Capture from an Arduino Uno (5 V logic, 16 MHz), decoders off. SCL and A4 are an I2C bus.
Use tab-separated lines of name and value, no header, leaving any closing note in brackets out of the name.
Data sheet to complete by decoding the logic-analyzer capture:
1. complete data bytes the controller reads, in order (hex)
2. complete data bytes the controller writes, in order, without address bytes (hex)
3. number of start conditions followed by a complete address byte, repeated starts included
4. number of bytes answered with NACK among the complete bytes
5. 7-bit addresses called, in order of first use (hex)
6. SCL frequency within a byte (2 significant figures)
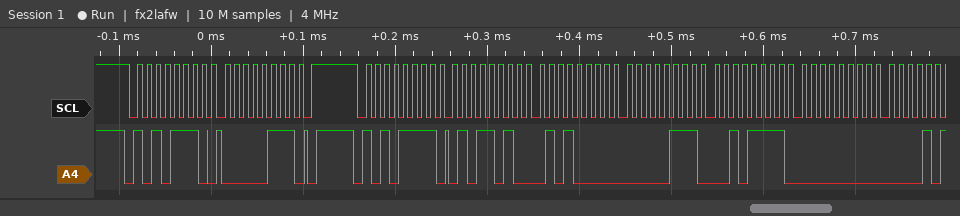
complete data bytes the controller reads, in order	5A 50 07 2F 00
complete data bytes the controller writes, in order, without address bytes	07
number of start conditions followed by a complete address byte, repeated starts included	2
number of bytes answered with NACK among the complete bytes	0
7-bit addresses called, in order of first use	0x57
SCL frequency within a byte	100 kHz
